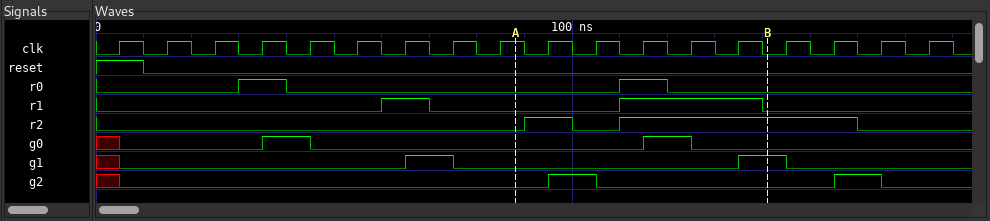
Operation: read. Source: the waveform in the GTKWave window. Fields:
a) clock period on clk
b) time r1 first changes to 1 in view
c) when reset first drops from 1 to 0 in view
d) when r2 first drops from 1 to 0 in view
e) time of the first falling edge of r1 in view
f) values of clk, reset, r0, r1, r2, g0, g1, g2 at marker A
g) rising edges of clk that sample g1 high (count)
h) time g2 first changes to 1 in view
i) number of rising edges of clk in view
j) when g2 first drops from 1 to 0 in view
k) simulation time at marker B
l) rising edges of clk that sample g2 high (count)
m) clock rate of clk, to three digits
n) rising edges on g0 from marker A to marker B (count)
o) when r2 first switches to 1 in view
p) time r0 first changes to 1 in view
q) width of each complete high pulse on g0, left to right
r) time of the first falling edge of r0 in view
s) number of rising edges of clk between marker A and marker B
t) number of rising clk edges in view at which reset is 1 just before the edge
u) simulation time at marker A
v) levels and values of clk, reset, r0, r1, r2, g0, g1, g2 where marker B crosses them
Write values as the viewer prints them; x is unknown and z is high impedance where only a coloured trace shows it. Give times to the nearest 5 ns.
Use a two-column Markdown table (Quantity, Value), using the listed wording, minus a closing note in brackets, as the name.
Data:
| Quantity | Value |
|---|---|
| clock period on clk | 10 ns |
| time r1 first changes to 1 in view | 60 ns |
| when reset first drops from 1 to 0 in view | 10 ns |
| when r2 first drops from 1 to 0 in view | 100 ns |
| time of the first falling edge of r1 in view | 70 ns |
| values of clk, reset, r0, r1, r2, g0, g1, g2 at marker A | clk=1, reset=0, r0=0, r1=0, r2=0, g0=0, g1=0, g2=0 |
| rising edges of clk that sample g1 high | 2 |
| time g2 first changes to 1 in view | 95 ns |
| number of rising edges of clk in view | 18 |
| when g2 first drops from 1 to 0 in view | 105 ns |
| simulation time at marker B | 140 ns |
| rising edges of clk that sample g2 high | 2 |
| clock rate of clk, to three digits | 100 MHz |
| rising edges on g0 from marker A to marker B | 1 |
| when r2 first switches to 1 in view | 90 ns |
| time r0 first changes to 1 in view | 30 ns |
| width of each complete high pulse on g0, left to right | 10 ns, 10 ns |
| time of the first falling edge of r0 in view | 40 ns |
| number of rising edges of clk between marker A and marker B | 5 |
| number of rising clk edges in view at which reset is 1 just before the edge | 1 |
| simulation time at marker A | 90 ns |
| levels and values of clk, reset, r0, r1, r2, g0, g1, g2 where marker B crosses them | clk=0, reset=0, r0=0, r1=0, r2=1, g0=0, g1=1, g2=0 |
